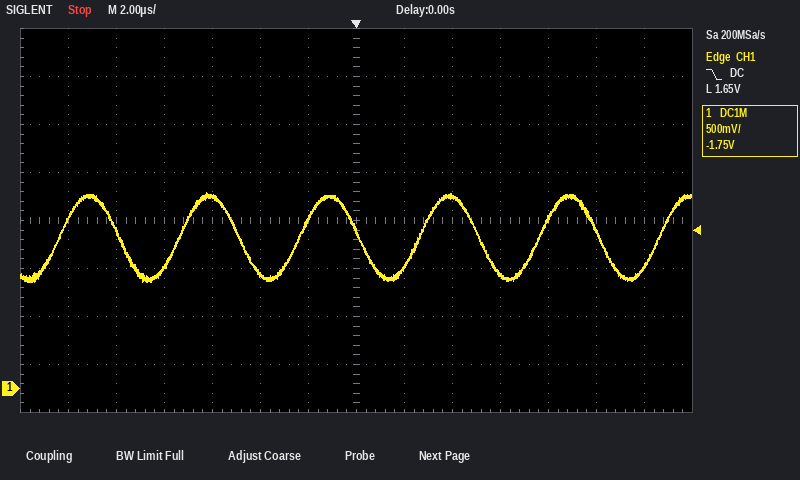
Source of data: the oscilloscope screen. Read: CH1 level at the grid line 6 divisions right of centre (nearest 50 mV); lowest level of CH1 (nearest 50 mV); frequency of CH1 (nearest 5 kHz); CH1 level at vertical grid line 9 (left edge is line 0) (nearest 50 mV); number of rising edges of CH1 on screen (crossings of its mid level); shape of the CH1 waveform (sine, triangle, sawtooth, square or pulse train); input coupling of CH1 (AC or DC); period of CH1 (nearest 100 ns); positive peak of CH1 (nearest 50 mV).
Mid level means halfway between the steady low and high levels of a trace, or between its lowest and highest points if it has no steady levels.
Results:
1.25 V
1.10 V
200 kHz
2.00 V
6
sine
DC
5.0 µs
2.05 V
